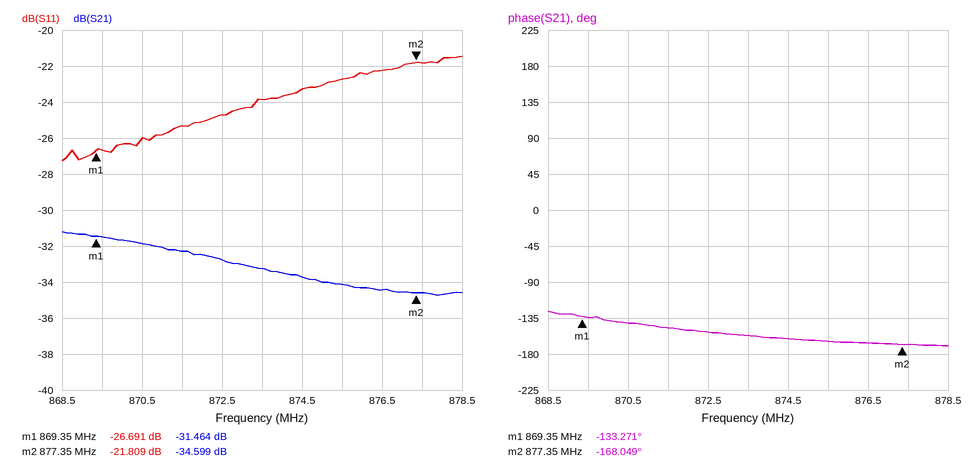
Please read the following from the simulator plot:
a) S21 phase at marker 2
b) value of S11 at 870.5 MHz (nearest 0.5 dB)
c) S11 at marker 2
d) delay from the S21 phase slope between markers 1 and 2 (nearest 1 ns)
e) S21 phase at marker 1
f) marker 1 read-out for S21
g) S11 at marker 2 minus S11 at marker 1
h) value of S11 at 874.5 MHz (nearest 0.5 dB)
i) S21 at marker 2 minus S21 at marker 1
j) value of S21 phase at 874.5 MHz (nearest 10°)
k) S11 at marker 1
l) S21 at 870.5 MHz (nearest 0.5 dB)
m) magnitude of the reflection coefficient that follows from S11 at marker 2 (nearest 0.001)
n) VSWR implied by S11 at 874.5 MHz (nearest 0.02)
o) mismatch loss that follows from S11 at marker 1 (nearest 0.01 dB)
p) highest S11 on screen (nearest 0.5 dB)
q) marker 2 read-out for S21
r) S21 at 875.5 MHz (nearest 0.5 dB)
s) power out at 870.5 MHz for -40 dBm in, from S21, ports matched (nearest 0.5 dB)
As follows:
-168.049°
-26.0 dB
-21.809 dB
12 ns
-133.271°
-31.464 dB
4.882 dB
-23.5 dB
-3.135 dB
-160°
-26.691 dB
-32.0 dB
0.081
1.14
0.01 dB
-21.5 dB
-34.599 dB
-34.0 dB
-72.0 dBm
